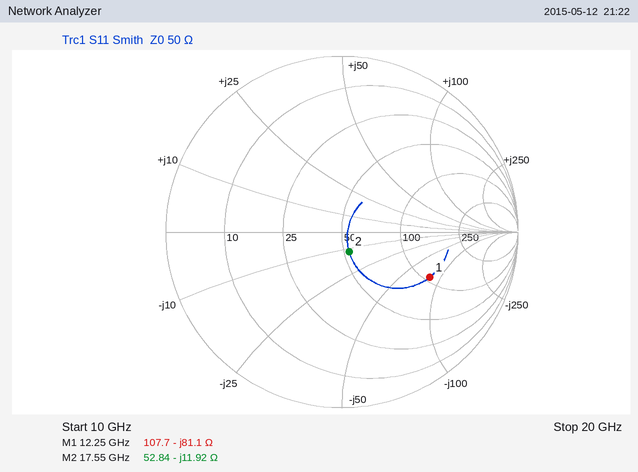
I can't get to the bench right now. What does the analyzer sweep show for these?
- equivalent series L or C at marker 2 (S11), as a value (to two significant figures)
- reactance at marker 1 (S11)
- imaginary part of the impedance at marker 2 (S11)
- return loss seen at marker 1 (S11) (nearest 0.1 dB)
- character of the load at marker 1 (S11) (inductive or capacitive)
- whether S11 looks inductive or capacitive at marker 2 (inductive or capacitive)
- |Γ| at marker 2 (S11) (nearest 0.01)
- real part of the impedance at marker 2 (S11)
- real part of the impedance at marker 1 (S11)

760 fF
-81.1 Ω
-11.92 Ω
5.0 dB
capacitive
capacitive
0.12
52.84 Ω
107.7 Ω
